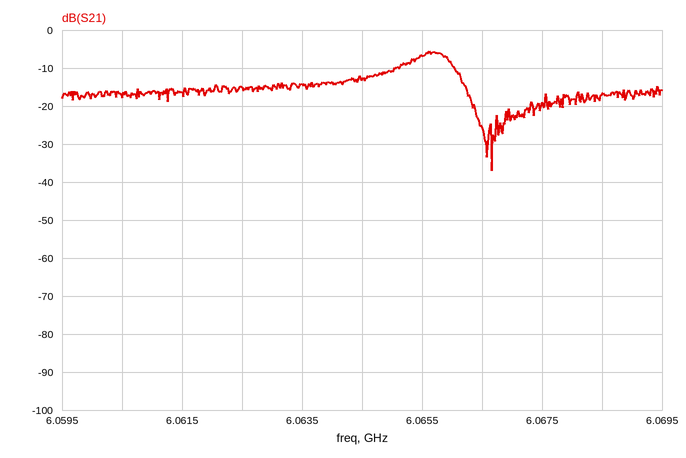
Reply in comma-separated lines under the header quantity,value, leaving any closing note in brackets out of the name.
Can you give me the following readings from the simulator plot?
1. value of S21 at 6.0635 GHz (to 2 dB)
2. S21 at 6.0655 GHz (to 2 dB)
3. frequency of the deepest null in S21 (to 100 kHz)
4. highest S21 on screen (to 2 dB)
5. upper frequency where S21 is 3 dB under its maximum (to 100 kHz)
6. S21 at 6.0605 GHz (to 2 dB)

quantity,value
value of S21 at 6.0635 GHz,-14 dB
S21 at 6.0655 GHz,-6 dB
frequency of the deepest null in S21,6.0667 GHz
highest S21 on screen,-6 dB
upper frequency where S21 is 3 dB under its maximum,6.0660 GHz
S21 at 6.0605 GHz,-18 dB
